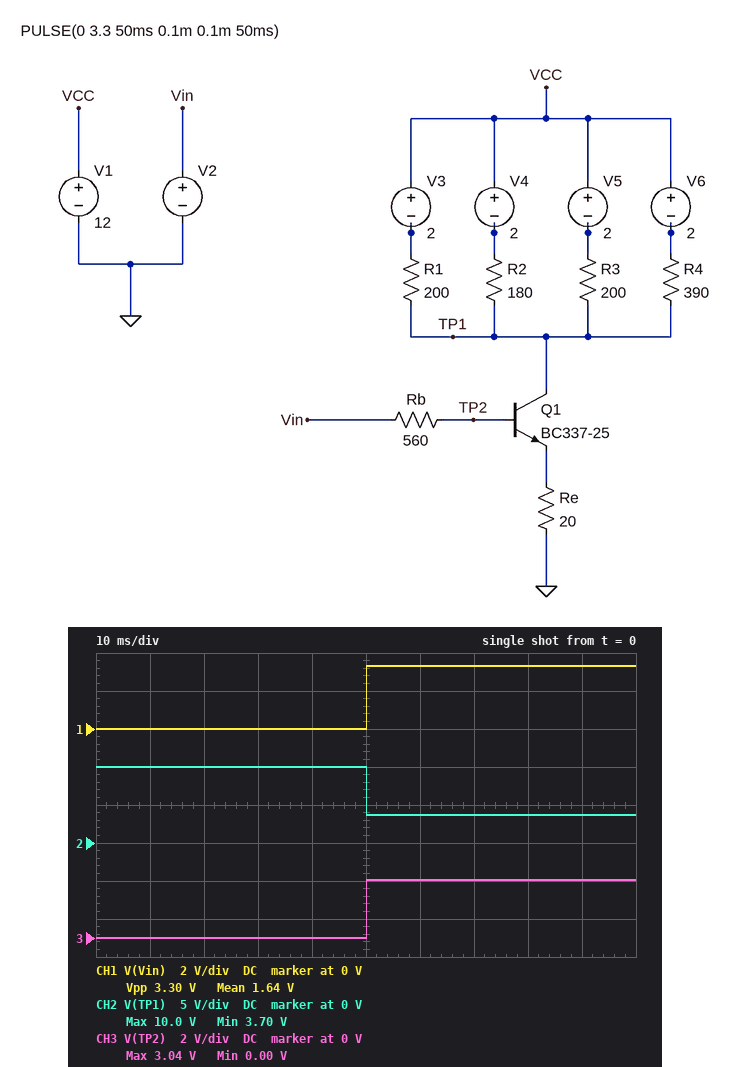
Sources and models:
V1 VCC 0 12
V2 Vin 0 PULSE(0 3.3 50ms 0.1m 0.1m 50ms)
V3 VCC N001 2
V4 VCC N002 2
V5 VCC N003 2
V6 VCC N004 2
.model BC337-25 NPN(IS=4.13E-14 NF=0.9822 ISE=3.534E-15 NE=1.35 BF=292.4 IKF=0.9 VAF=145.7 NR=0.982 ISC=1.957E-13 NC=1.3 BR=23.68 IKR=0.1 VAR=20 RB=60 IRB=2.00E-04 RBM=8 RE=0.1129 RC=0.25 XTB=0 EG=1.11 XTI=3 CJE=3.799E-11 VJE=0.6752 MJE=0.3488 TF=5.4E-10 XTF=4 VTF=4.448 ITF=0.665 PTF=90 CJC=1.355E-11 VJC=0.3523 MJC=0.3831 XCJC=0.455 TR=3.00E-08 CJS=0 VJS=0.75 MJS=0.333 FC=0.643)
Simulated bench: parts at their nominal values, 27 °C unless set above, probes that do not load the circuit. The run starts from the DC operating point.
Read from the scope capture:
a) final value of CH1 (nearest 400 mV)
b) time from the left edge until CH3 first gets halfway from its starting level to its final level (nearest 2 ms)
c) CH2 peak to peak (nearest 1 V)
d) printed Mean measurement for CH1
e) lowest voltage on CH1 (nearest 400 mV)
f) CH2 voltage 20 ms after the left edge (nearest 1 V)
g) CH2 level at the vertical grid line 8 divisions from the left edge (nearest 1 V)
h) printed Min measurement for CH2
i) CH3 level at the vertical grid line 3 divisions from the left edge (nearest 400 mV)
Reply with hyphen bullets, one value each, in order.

- 3.2 V
- 50 ms
- 6 V
- 1.64 V
- 0 V
- 10 V
- 4 V
- 3.70 V
- 0 V
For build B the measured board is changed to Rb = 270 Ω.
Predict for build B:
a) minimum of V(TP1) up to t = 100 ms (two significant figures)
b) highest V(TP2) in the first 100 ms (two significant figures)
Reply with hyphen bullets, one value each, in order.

- 3.4 V
- 3.2 V
